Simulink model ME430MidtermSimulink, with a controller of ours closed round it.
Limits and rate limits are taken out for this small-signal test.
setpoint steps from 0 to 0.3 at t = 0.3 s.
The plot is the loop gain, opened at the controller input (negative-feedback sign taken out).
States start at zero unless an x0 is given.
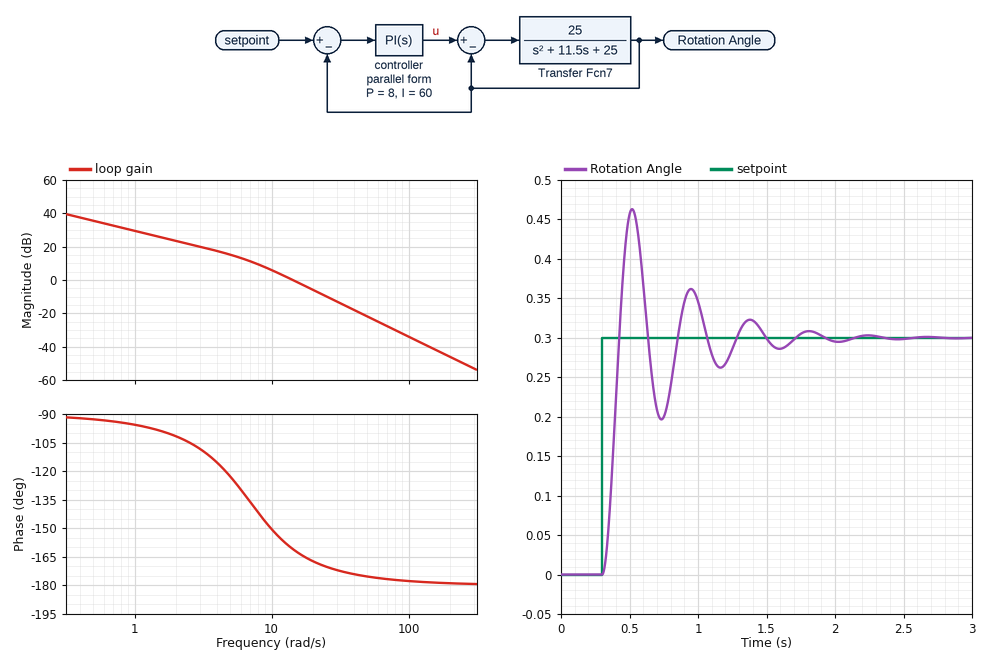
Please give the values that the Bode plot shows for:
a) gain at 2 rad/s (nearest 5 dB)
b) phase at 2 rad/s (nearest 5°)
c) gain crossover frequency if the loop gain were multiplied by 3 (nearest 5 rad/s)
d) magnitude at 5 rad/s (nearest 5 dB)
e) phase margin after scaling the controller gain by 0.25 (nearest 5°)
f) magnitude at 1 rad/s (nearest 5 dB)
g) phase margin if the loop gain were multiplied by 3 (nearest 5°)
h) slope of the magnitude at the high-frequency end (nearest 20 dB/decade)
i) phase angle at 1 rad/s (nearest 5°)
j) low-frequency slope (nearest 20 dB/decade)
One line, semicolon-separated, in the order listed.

25 dB; -100°; 25 rad/s; 15 dB; 45°; 30 dB; 10°; -40 dB/decade; -95°; -20 dB/decade
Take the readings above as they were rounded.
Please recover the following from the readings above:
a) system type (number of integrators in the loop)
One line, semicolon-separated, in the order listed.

1
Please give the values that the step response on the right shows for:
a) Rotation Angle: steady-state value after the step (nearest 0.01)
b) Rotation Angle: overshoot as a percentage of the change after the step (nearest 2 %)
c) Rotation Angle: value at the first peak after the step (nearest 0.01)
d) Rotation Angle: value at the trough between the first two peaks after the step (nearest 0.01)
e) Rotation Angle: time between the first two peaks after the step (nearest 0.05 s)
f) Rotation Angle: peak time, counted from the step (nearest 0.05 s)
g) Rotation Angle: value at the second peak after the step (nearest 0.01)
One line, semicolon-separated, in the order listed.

0.30; 54 %; 0.46; 0.20; 0.45 s; 0.20 s; 0.36
